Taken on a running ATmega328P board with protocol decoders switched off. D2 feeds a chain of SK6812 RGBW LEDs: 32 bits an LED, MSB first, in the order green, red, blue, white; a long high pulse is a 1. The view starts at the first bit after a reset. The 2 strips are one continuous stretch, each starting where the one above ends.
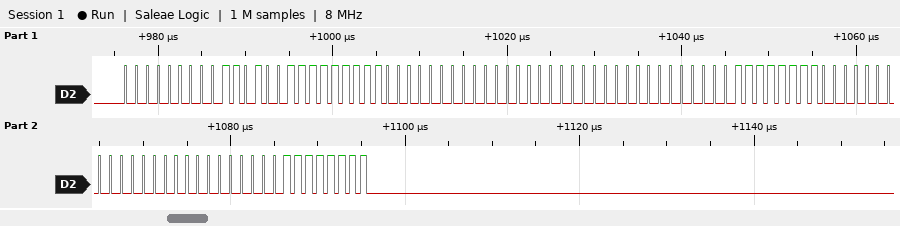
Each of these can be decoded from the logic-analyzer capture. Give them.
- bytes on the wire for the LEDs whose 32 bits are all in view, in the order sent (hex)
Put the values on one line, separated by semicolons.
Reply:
00 69 FF 00 00 00 00 FF 00 00 00 FF
